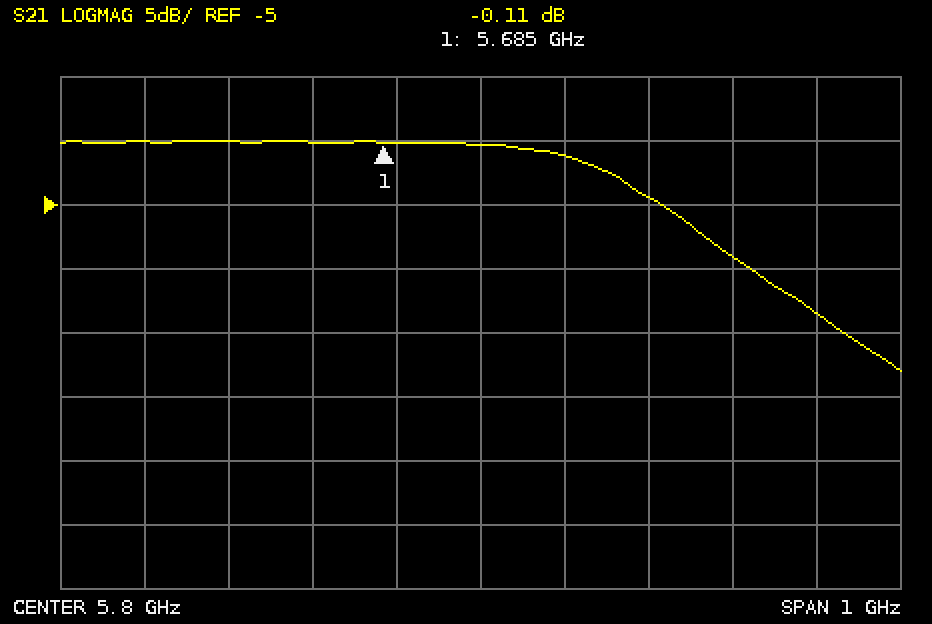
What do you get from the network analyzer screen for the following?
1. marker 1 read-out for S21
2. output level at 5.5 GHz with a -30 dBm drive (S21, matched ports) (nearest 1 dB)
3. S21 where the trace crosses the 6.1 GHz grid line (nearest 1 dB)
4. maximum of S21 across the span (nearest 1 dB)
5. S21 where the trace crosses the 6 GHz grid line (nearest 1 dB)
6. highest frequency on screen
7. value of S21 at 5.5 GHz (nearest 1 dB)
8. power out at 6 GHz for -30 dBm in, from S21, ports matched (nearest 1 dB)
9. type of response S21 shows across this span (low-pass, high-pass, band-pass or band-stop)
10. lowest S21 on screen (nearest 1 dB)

-0.11 dB
-30 dBm
-9 dB
0 dB
-4 dB
6.3 GHz
0 dB
-34 dBm
low-pass
-18 dB
